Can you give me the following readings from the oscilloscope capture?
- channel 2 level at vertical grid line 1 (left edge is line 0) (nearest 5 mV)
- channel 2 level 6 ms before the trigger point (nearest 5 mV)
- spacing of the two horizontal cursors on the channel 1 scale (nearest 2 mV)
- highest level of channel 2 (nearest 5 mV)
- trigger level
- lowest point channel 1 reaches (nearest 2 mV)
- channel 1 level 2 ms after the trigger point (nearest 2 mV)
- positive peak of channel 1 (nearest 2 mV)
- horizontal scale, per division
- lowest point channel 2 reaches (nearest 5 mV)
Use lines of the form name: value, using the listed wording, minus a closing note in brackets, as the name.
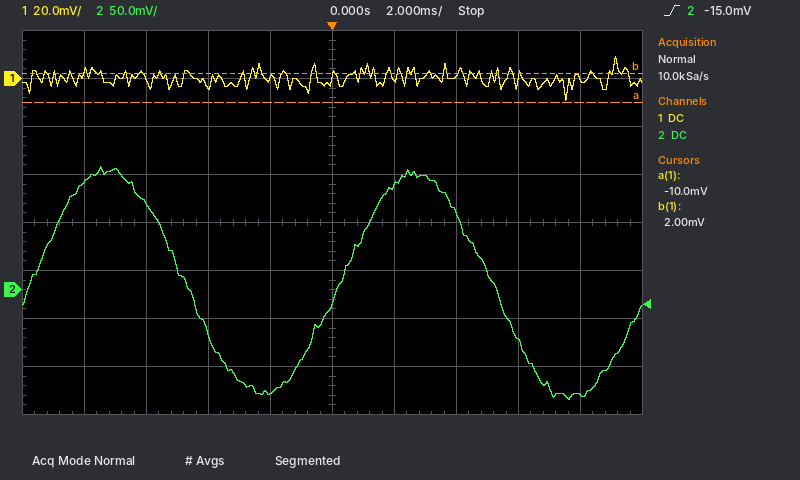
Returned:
channel 2 level at vertical grid line 1 (left edge is line 0): 110 mV
channel 2 level 6 ms before the trigger point: 90 mV
spacing of the two horizontal cursors on the channel 1 scale: 12 mV
highest level of channel 2: 130 mV
trigger level: -15.0 mV
lowest point channel 1 reaches: -10 mV
channel 1 level 2 ms after the trigger point: 0 mV
positive peak of channel 1: 10 mV
horizontal scale, per division: 2 ms
lowest point channel 2 reaches: -115 mV
